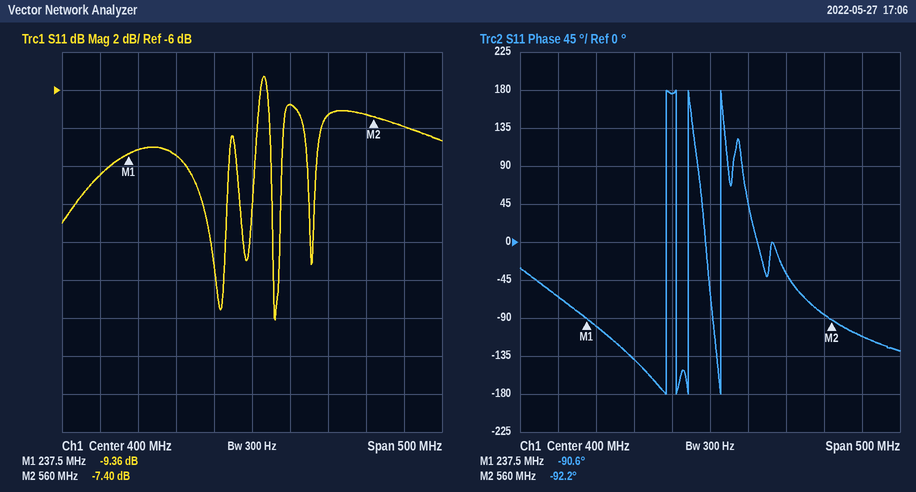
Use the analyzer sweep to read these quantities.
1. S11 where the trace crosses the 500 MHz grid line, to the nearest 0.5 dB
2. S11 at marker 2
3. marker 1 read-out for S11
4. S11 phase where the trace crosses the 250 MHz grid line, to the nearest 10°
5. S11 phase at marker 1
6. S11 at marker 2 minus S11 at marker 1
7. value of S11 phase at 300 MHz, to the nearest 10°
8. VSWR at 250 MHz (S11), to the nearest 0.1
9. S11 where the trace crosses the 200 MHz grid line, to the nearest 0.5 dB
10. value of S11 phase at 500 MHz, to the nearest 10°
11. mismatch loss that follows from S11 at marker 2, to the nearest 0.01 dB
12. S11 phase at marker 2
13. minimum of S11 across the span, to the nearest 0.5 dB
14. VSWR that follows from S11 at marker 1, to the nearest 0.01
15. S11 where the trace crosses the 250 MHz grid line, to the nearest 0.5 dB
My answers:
-7.5 dB
-7.40 dB
-9.36 dB
-100°
-90.6°
1.96 dB
-140°
2.1
-10.5 dB
-40°
0.87 dB
-92.2°
-18.0 dB
2.03
-9.0 dB
